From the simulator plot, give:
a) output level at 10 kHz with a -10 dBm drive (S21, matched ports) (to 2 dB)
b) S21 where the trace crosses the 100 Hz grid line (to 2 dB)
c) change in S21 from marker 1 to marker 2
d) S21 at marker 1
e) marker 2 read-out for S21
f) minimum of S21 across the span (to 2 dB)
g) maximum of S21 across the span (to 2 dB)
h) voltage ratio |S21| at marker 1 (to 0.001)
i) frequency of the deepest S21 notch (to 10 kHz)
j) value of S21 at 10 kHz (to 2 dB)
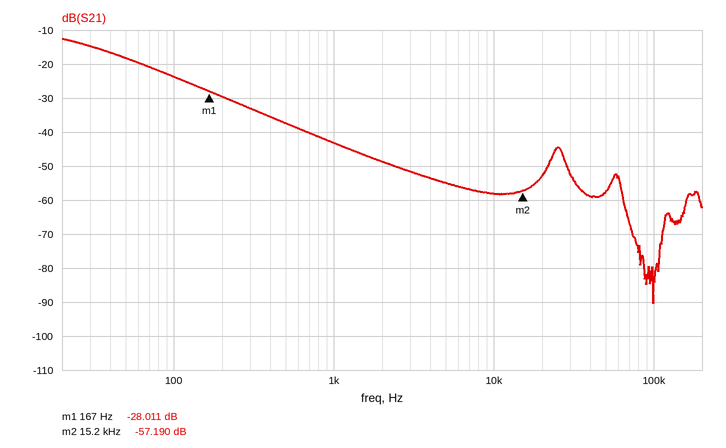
-68 dBm
-24 dB
-29.179 dB
-28.011 dB
-57.190 dB
-90 dB
-12 dB
0.040
100 kHz
-58 dB
